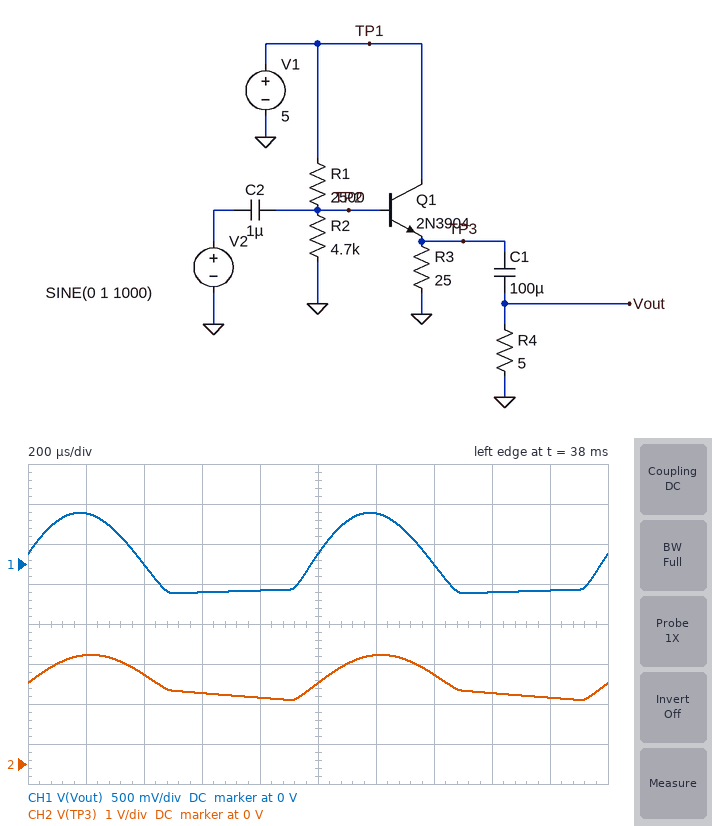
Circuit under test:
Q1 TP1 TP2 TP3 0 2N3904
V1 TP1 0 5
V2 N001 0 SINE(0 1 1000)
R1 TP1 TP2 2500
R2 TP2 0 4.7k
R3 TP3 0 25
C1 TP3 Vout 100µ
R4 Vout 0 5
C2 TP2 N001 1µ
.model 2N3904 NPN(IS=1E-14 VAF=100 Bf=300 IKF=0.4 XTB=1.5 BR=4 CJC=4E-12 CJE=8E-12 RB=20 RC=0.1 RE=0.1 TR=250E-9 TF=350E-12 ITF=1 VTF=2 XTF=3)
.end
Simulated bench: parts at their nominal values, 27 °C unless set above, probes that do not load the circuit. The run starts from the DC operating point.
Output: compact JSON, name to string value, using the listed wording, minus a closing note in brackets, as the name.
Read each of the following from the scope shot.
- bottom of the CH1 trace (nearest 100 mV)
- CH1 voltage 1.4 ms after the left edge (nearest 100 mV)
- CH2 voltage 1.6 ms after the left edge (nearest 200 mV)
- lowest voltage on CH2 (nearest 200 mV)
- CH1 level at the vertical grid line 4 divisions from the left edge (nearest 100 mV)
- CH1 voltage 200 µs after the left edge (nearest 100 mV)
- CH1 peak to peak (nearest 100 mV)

{"bottom of the CH1 trace": "-400 mV", "CH1 voltage 1.4 ms after the left edge": "0 V", "CH2 voltage 1.6 ms after the left edge": "1.8 V", "lowest voltage on CH2": "1.6 V", "CH1 level at the vertical grid line 4 divisions from the left edge": "-300 mV", "CH1 voltage 200 µs after the left edge": "600 mV", "CH1 peak to peak": "1.0 V"}
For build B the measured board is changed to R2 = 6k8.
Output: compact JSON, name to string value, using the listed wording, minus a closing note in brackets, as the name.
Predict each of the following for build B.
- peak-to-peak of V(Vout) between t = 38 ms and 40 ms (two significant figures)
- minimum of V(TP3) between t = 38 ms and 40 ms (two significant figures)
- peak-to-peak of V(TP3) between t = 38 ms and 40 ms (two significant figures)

{"peak-to-peak of V(Vout) between t = 38 ms and 40 ms": "1.1 V", "minimum of V(TP3) between t = 38 ms and 40 ms": "1.8 V", "peak-to-peak of V(TP3) between t = 38 ms and 40 ms": "1.2 V"}
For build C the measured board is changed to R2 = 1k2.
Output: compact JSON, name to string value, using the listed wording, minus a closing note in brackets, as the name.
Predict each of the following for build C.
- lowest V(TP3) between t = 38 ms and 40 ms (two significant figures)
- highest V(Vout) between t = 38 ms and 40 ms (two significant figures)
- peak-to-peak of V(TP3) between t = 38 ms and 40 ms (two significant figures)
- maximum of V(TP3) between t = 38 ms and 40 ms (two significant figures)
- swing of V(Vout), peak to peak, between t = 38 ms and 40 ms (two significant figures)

{"lowest V(TP3) between t = 38 ms and 40 ms": "850 mV", "highest V(Vout) between t = 38 ms and 40 ms": "480 mV", "peak-to-peak of V(TP3) between t = 38 ms and 40 ms": "760 mV", "maximum of V(TP3) between t = 38 ms and 40 ms": "1.6 V", "swing of V(Vout), peak to peak, between t = 38 ms and 40 ms": "680 mV"}
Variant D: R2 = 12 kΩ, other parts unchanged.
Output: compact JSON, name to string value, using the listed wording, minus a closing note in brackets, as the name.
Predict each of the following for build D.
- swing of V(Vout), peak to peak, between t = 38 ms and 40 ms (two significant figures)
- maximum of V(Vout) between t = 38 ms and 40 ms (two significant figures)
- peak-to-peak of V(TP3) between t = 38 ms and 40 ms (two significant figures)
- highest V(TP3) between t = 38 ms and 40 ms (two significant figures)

{"swing of V(Vout), peak to peak, between t = 38 ms and 40 ms": "1.1 V", "maximum of V(Vout) between t = 38 ms and 40 ms": "690 mV", "peak-to-peak of V(TP3) between t = 38 ms and 40 ms": "1.3 V", "highest V(TP3) between t = 38 ms and 40 ms": "3.2 V"}
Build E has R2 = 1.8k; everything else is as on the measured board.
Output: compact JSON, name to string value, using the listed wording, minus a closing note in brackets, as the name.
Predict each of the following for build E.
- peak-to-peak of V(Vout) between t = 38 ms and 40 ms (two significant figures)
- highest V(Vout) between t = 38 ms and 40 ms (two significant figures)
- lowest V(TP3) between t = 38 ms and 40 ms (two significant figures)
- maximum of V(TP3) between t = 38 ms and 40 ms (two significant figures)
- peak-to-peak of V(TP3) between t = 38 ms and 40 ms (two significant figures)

{"peak-to-peak of V(Vout) between t = 38 ms and 40 ms": "790 mV", "highest V(Vout) between t = 38 ms and 40 ms": "540 mV", "lowest V(TP3) between t = 38 ms and 40 ms": "1.1 V", "maximum of V(TP3) between t = 38 ms and 40 ms": "2.0 V", "peak-to-peak of V(TP3) between t = 38 ms and 40 ms": "880 mV"}
